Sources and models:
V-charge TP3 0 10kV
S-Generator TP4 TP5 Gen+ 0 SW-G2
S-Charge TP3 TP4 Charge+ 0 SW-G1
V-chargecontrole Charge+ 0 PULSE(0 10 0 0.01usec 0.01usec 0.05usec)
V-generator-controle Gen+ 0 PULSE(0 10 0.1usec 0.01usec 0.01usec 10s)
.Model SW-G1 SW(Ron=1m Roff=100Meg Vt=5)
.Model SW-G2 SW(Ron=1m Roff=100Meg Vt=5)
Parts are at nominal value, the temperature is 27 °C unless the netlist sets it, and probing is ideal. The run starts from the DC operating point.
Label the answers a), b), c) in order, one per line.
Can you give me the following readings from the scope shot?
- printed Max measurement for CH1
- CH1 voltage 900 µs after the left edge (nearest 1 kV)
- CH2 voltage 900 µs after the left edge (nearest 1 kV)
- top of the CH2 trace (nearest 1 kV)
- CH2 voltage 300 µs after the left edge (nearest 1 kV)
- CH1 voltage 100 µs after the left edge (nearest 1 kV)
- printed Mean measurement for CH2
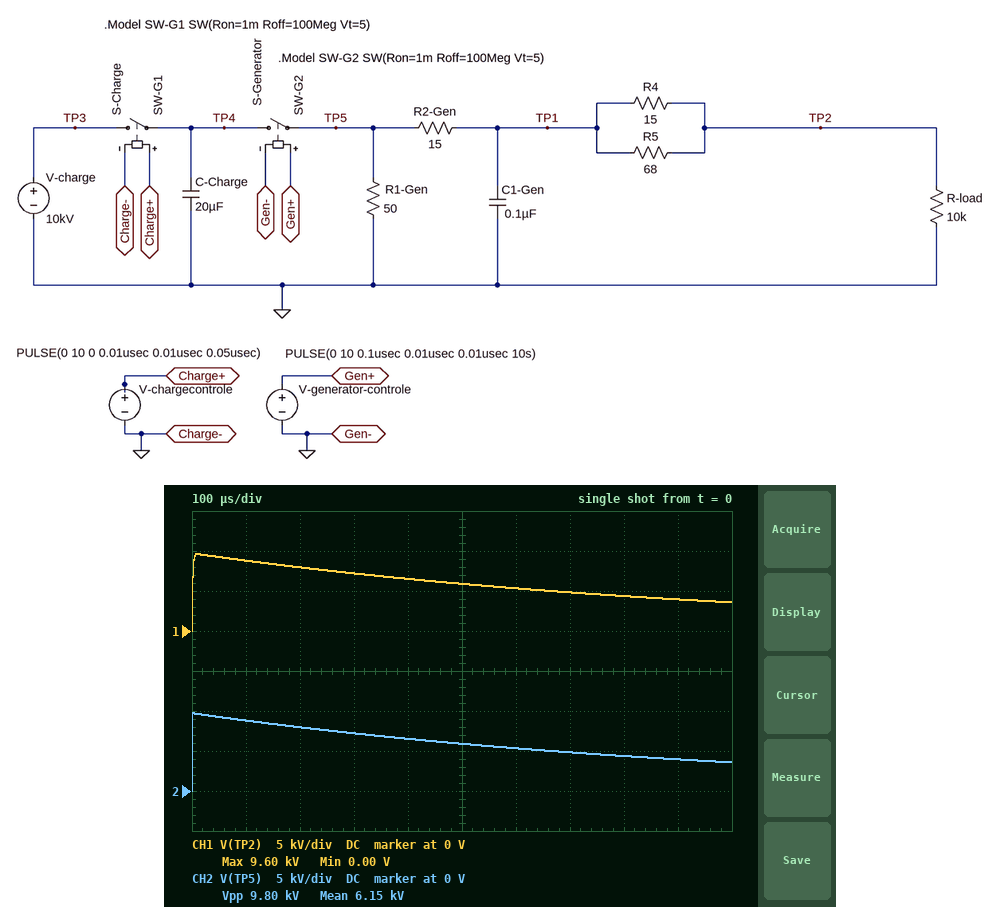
a) 9.60 kV
b) 4 kV
c) 4 kV
d) 10 kV
e) 7 kV
f) 9 kV
g) 6.15 kV
